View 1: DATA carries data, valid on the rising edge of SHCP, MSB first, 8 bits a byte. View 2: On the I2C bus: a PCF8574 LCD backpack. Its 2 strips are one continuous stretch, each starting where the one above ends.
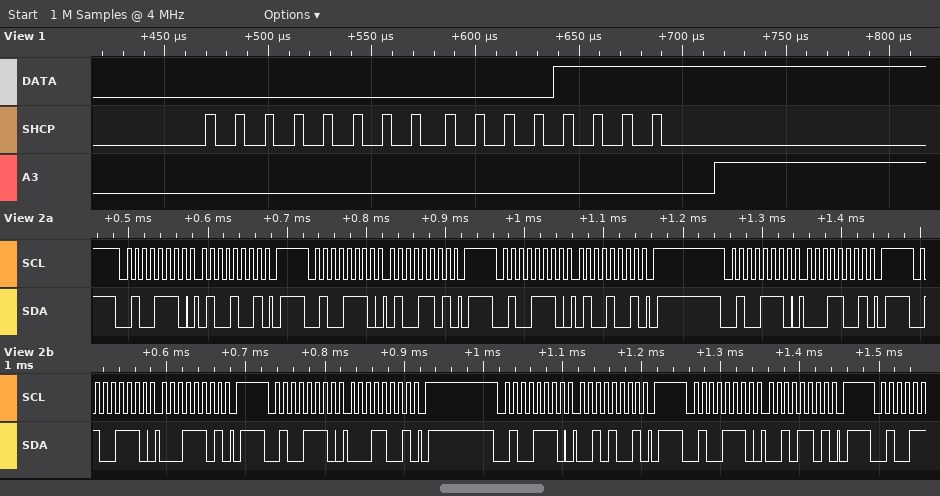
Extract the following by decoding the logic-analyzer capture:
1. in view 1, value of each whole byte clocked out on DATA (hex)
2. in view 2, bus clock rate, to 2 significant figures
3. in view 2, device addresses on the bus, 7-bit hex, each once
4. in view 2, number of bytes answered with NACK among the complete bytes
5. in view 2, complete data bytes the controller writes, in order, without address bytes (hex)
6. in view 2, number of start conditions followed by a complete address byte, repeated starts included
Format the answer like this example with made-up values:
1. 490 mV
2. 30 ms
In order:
1. 00 0F
2. 100 kHz
3. 0x27
4. 0
5. 49 4D 49 19 1D 19 29 2D
6. 8
